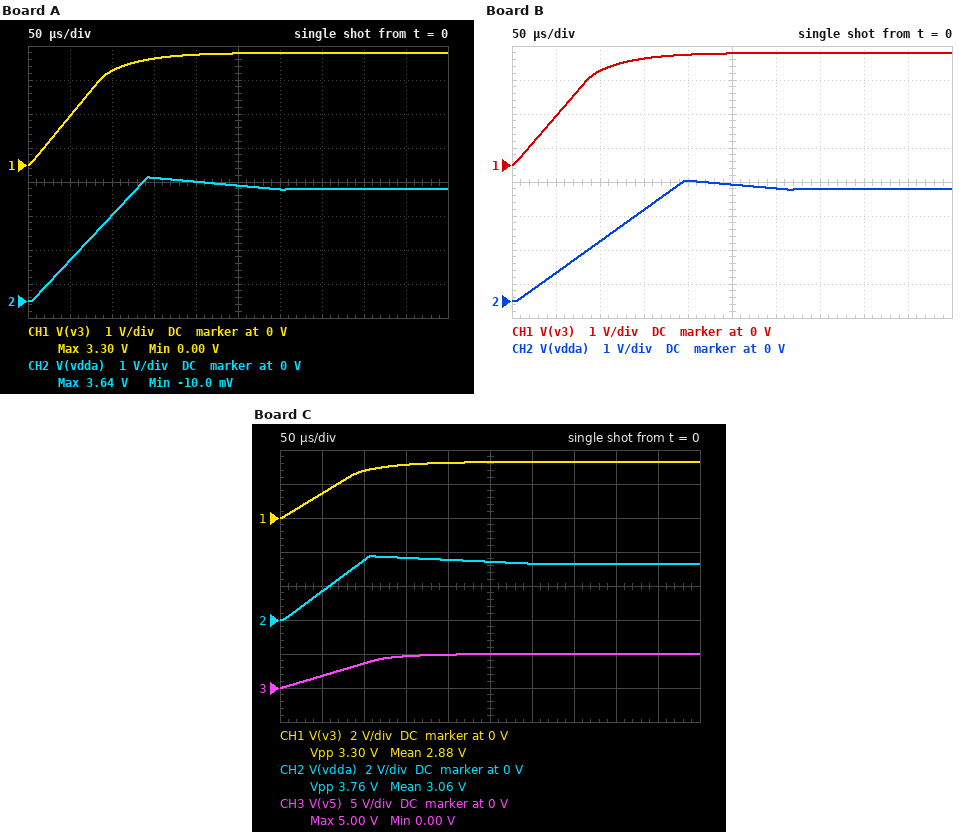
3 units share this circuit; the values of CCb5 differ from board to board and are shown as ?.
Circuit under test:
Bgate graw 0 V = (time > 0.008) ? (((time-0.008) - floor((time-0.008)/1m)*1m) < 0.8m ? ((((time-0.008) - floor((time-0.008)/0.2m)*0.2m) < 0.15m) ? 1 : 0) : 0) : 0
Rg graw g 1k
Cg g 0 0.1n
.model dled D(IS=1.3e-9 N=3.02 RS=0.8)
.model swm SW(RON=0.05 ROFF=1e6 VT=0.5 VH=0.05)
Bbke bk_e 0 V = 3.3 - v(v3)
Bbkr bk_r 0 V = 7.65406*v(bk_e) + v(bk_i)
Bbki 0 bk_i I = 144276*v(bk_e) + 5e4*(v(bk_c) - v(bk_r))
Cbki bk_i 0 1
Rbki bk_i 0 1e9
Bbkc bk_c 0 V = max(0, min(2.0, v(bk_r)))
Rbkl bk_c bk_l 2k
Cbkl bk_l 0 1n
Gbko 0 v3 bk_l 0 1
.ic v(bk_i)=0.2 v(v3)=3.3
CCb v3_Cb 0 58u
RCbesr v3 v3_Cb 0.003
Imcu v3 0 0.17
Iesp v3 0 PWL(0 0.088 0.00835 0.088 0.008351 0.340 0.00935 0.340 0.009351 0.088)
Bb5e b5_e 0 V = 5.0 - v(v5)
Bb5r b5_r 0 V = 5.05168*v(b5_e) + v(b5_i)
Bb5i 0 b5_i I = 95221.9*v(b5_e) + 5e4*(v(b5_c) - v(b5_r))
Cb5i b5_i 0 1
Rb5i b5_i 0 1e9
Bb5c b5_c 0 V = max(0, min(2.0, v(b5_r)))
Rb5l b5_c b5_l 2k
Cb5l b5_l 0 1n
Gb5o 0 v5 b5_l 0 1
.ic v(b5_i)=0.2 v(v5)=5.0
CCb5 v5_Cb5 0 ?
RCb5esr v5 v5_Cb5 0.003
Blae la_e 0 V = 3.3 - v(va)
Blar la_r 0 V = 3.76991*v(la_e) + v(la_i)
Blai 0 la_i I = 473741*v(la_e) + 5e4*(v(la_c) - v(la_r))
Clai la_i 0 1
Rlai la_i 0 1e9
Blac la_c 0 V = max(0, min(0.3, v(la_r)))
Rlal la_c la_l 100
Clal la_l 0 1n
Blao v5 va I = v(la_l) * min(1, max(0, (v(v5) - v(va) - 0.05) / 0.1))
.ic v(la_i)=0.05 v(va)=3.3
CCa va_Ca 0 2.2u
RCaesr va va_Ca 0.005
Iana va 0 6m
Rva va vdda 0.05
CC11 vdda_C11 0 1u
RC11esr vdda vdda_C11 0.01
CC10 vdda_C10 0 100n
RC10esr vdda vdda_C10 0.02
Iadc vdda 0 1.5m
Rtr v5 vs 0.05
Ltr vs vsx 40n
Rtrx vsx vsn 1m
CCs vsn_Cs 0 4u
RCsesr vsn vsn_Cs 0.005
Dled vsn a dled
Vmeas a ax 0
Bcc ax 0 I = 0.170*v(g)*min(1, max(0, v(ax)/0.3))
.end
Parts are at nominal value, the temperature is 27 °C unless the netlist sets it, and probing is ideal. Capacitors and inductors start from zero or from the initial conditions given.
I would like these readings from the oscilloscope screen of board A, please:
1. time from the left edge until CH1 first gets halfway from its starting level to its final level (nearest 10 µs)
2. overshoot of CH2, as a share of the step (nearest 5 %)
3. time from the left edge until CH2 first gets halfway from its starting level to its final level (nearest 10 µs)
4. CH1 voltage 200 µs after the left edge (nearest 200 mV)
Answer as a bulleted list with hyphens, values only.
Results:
- 60 µs
- 10 %
- 70 µs
- 3.2 V
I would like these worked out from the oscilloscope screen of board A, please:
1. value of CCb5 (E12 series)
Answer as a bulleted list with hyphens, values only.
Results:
- 68 µF
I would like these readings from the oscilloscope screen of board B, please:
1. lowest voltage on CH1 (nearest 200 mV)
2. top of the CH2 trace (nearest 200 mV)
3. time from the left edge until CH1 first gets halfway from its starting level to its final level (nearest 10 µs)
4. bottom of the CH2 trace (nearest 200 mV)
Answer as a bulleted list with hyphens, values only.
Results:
- 0 V
- 3.6 V
- 60 µs
- 0 V
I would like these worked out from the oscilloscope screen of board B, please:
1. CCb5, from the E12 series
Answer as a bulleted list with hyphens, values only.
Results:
- 100 µF
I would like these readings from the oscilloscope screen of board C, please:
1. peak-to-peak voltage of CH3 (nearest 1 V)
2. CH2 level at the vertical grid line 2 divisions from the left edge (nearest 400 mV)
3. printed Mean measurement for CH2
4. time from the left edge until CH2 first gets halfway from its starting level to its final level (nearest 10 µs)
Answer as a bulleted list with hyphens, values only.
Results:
- 5 V
- 3.6 V
- 3.06 V
- 50 µs
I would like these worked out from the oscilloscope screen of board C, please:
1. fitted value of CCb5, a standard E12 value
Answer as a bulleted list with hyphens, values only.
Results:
- 47 µF
